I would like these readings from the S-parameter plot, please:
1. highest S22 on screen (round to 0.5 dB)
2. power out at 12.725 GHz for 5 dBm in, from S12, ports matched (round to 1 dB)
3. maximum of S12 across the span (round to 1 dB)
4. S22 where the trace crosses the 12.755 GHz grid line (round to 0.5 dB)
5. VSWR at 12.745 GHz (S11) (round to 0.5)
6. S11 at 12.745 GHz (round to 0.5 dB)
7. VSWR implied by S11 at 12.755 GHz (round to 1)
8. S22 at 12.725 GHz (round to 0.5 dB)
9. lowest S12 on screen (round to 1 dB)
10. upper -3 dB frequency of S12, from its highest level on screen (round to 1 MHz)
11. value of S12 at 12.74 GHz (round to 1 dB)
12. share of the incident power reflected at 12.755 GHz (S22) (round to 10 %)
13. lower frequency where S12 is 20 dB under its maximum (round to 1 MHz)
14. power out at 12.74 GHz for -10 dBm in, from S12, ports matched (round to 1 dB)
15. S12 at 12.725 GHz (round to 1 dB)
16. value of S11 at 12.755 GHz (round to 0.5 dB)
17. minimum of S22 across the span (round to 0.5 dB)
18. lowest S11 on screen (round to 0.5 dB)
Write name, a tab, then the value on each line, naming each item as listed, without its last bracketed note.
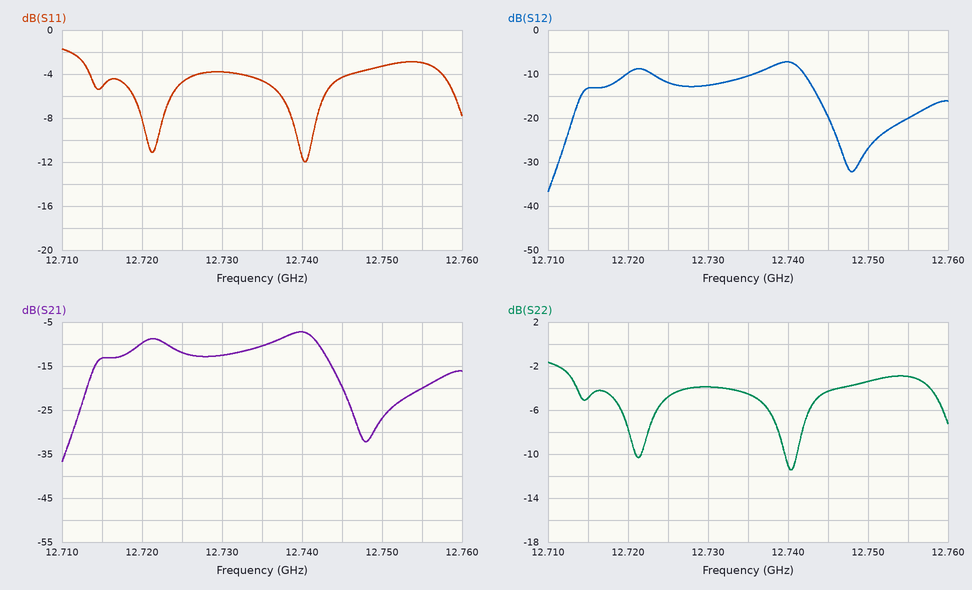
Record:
highest S22 on screen	-1.5 dB
power out at 12.725 GHz for 5 dBm in, from S12, ports matched	-7 dBm
maximum of S12 across the span	-7 dB
S22 where the trace crosses the 12.755 GHz grid line	-3.0 dB
VSWR at 12.745 GHz (S11)	4.0
S11 at 12.745 GHz	-4.5 dB
VSWR implied by S11 at 12.755 GHz	6
S22 at 12.725 GHz	-5.0 dB
lowest S12 on screen	-37 dB
upper -3 dB frequency of S12, from its highest level on screen	12.742 GHz
value of S12 at 12.74 GHz	-7 dB
share of the incident power reflected at 12.755 GHz (S22)	50 %
lower frequency where S12 is 20 dB under its maximum	12.712 GHz
power out at 12.74 GHz for -10 dBm in, from S12, ports matched	-17 dBm
S12 at 12.725 GHz	-12 dB
value of S11 at 12.755 GHz	-3.0 dB
minimum of S22 across the span	-11.5 dB
lowest S11 on screen	-12.0 dB
